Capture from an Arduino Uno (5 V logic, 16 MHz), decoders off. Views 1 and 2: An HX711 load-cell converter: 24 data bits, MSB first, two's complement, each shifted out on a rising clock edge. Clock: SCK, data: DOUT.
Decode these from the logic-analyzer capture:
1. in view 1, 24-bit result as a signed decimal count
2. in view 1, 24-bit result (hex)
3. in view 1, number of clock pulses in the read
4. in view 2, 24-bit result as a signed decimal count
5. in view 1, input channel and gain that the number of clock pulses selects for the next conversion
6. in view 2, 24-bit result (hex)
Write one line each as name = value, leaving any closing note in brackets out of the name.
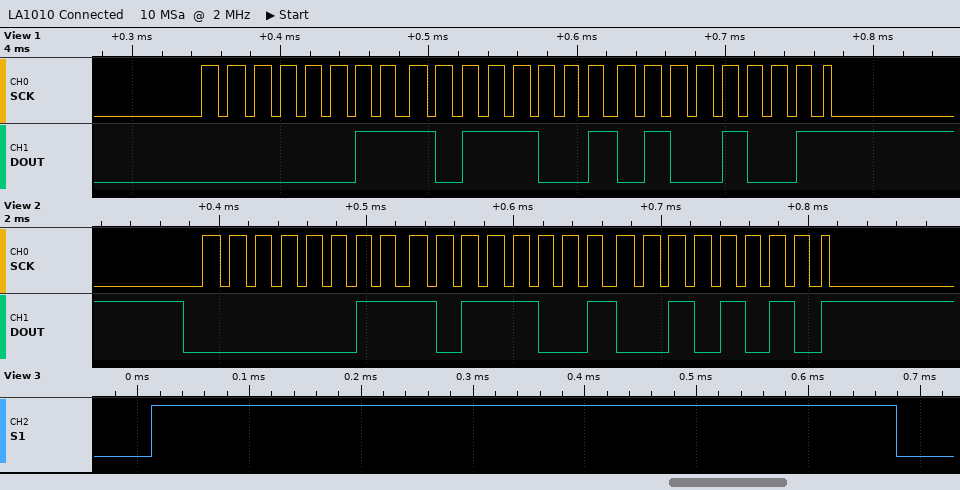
in view 1, 24-bit result as a signed decimal count = 244041
in view 1, 24-bit result = 0x03B949
in view 1, number of clock pulses in the read = 25
in view 2, 24-bit result as a signed decimal count = 244010
in view 1, input channel and gain that the number of clock pulses selects for the next conversion = channel A, gain 128
in view 2, 24-bit result = 0x03B92A
